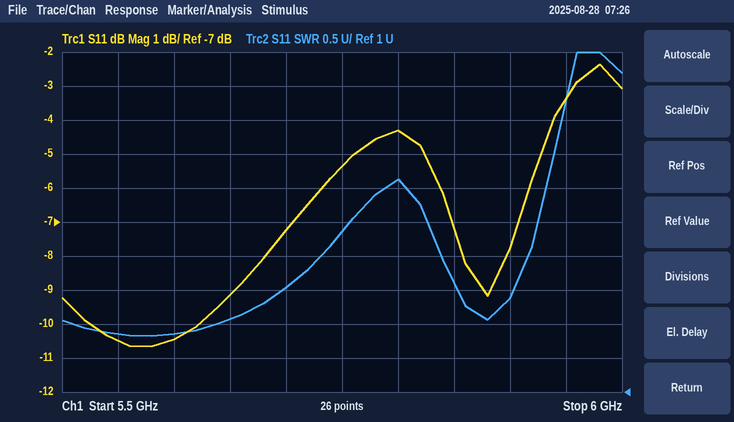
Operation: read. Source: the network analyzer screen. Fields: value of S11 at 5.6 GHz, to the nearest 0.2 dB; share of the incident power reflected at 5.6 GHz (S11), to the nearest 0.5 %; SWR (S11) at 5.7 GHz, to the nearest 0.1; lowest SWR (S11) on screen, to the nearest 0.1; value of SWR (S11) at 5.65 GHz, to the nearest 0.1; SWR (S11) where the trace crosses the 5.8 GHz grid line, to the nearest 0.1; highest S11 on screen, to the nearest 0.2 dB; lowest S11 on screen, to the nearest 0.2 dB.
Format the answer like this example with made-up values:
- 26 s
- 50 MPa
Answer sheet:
- -10.4 dB
- 9.0 %
- 2.5
- 1.8
- 2.1
- 4.1
- -2.4 dB
- -10.6 dB
